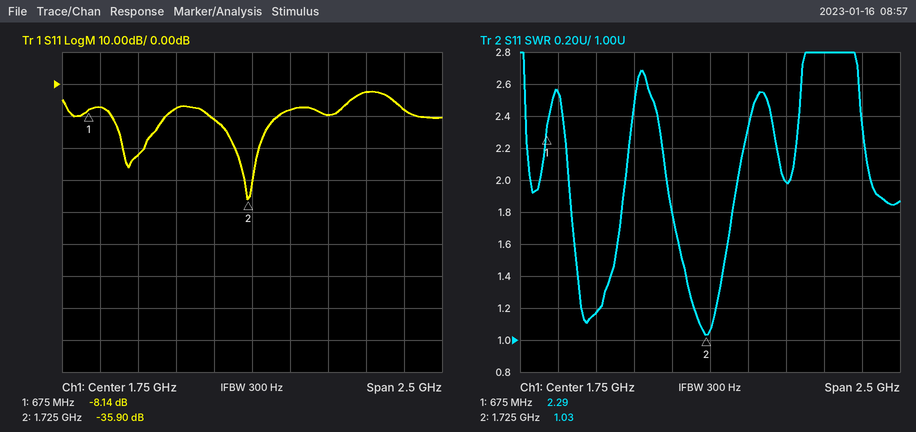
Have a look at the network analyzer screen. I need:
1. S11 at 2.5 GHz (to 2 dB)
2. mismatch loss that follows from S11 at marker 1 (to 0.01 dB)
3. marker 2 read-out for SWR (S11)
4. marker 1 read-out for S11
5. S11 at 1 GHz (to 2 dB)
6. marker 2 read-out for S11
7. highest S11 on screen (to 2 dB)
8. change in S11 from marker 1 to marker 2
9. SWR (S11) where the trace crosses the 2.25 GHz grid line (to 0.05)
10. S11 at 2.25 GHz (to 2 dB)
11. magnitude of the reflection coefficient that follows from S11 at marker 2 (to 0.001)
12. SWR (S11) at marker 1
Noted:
-2 dB
0.72 dB
1.03
-8.14 dB
-22 dB
-35.90 dB
-2 dB
-27.76 dB
2.00
-10 dB
0.016
2.29
